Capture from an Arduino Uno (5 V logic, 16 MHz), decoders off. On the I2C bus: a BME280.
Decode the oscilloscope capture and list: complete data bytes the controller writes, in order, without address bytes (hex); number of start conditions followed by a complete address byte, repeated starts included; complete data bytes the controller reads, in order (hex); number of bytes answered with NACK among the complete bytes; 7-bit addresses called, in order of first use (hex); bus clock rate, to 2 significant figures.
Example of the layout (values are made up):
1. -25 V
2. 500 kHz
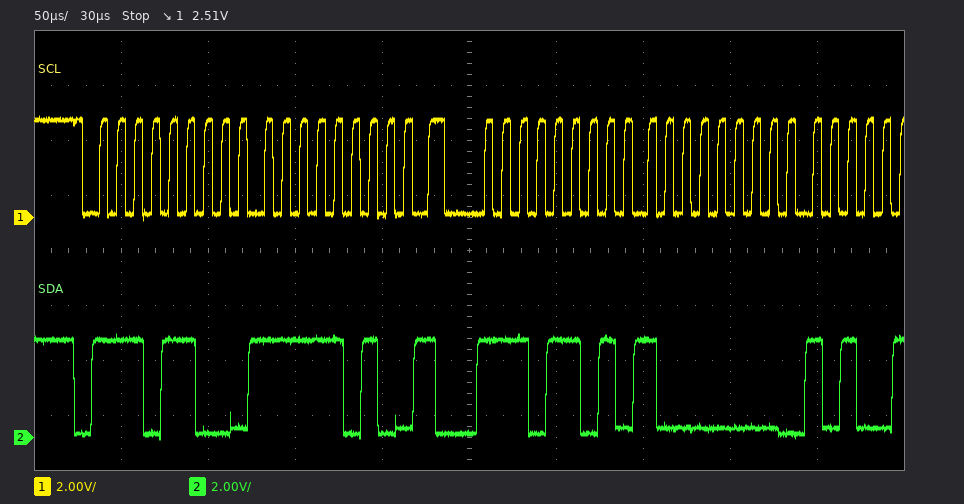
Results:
1. FA
2. 2
3. 80
4. 0
5. 0x76
6. 100 kHz
